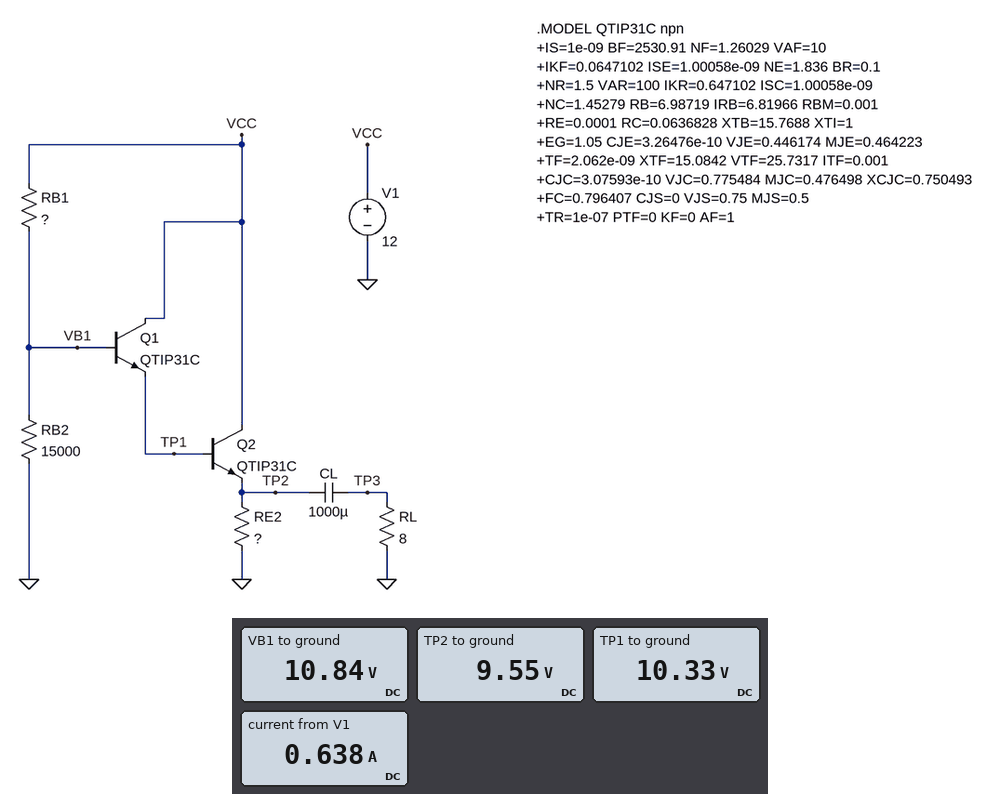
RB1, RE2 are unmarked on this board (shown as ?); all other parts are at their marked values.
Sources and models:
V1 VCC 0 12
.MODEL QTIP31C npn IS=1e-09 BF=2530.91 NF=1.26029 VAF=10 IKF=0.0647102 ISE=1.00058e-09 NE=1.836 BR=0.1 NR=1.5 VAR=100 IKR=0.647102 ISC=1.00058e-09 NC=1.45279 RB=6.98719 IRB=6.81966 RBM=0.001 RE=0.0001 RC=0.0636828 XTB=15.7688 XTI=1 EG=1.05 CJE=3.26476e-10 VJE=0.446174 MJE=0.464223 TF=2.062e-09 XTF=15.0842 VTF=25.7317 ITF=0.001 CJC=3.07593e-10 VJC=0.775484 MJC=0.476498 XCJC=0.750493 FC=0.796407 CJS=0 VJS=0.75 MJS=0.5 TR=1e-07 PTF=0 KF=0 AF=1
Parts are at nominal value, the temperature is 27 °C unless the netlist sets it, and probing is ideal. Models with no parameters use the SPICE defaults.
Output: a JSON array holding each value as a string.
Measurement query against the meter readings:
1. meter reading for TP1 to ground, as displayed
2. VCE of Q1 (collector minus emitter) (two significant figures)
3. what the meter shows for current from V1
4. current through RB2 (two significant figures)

["10.33 V", "1.7 V", "0.638 A", "720 µA"]
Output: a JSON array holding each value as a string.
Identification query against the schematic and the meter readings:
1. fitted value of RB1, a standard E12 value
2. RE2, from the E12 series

["1.5 kΩ", "15 Ω"]
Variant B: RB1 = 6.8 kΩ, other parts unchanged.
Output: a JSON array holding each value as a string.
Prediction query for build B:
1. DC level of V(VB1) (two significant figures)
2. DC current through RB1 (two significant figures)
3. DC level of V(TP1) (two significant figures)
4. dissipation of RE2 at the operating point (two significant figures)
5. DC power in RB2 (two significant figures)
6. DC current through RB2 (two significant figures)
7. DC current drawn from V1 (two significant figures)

["8.1 V", "570 µA", "7.7 V", "3.2 W", "4.4 mW", "540 µA", "460 mA"]
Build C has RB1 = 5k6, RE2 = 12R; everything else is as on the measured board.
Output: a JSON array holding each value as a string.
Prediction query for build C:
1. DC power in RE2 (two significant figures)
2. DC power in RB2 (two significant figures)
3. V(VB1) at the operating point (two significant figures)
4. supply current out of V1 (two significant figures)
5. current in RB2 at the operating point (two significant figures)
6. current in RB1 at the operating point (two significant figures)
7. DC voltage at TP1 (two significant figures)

["4.5 W", "4.9 mW", "8.6 V", "610 mA", "570 µA", "610 µA", "8.1 V"]
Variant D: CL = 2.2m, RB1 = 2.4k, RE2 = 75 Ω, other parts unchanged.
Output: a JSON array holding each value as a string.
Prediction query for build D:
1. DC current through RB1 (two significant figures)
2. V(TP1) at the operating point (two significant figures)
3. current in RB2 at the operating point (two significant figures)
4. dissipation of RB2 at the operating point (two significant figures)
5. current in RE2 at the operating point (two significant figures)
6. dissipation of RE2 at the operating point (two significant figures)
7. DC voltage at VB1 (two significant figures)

["700 µA", "9.9 V", "690 µA", "7.1 mW", "120 mA", "1.1 W", "10 V"]
